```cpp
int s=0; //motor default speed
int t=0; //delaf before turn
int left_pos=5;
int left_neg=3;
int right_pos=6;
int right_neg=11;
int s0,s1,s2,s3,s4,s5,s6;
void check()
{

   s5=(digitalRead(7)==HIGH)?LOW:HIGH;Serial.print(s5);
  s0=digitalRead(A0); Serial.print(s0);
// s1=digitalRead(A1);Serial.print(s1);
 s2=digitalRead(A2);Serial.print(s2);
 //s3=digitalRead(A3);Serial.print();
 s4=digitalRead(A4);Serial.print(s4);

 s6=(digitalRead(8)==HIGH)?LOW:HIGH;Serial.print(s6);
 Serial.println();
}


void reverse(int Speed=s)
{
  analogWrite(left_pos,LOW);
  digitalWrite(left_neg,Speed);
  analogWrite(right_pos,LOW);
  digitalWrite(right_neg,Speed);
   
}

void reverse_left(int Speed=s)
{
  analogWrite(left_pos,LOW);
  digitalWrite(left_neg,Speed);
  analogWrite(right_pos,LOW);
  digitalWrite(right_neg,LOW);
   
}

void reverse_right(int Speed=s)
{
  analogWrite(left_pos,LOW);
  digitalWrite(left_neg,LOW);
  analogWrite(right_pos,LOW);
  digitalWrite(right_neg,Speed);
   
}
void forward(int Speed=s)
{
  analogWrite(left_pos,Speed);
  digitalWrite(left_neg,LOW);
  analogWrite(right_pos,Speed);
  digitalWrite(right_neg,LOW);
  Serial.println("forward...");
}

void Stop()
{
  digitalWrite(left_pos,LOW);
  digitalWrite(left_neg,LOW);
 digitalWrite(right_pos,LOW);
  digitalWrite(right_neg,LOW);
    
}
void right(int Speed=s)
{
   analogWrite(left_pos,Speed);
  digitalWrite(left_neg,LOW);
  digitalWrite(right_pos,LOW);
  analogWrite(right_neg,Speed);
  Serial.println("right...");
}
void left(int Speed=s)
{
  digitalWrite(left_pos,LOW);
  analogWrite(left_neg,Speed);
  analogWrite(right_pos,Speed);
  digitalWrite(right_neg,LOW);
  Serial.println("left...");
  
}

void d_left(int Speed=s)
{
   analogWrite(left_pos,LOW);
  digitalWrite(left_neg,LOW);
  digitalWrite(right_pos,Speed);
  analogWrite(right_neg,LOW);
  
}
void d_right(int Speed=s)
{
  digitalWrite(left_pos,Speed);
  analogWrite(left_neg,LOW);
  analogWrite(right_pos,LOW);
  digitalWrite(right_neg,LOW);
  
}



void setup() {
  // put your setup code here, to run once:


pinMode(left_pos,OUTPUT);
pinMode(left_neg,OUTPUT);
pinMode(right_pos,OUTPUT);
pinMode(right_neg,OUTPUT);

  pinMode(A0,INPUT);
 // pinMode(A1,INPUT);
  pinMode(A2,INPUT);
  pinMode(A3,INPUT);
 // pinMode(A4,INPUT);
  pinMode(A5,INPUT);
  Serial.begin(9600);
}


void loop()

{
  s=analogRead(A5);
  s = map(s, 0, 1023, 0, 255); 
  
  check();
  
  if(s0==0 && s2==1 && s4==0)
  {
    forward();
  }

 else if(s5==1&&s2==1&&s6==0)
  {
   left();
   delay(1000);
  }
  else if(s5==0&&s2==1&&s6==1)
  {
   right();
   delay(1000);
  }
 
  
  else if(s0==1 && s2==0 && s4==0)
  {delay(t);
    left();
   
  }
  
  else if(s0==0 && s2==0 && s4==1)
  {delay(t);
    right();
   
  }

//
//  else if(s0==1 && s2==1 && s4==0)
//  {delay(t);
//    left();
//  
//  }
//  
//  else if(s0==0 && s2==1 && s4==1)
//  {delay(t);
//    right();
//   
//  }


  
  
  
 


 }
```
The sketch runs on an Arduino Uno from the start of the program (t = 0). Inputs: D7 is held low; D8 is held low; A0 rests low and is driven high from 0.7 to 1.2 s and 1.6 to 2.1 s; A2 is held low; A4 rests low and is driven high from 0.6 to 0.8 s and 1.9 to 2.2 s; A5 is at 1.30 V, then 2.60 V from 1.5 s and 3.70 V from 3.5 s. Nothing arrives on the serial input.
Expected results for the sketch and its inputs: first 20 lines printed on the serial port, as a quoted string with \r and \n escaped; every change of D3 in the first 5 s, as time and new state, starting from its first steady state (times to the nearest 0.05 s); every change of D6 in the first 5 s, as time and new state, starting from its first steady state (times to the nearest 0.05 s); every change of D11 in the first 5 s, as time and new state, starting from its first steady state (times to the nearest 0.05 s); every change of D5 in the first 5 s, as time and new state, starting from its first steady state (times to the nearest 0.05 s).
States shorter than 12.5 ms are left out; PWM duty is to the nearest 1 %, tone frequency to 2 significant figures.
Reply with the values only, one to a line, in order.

"10001\r\n10001\r\n10001\r\n10001\r\n10001\r\n10001\r\n10001\r\n10001\r\n10001\r\n10001\r\n10001\r\n10001\r\n10001\r\n10001\r\n10001\r\n10001\r\n10001\r\n10001\r\n10001\r\n10001\r\n"
0 s low; 0.8 s PWM 26 %; 1.6 s PWM 52 %; 2.1 s low
0 s low; 0.8 s PWM 26 %; 1.6 s PWM 52 %; 2.1 s low
0 s low; 0.6 s PWM 26 %; 0.8 s low; 2.1 s PWM 52 %
0 s low; 0.6 s PWM 26 %; 0.8 s low; 2.1 s PWM 52 %
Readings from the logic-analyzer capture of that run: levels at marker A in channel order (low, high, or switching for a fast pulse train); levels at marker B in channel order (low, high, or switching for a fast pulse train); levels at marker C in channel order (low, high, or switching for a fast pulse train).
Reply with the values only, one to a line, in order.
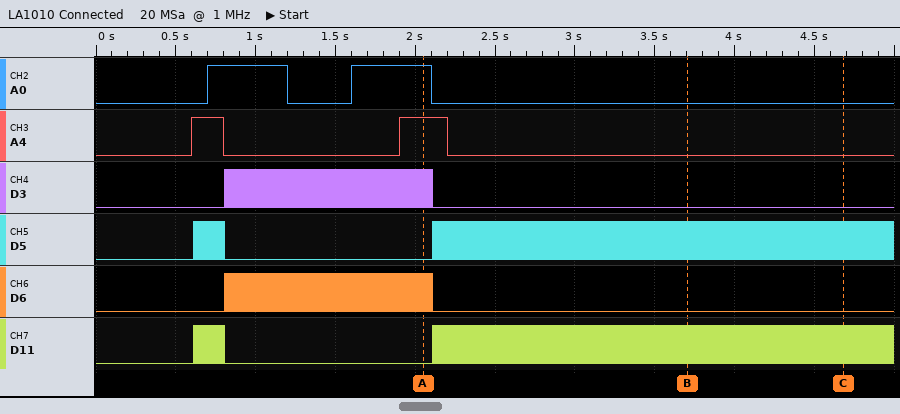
A0 high, A4 high, D3 switching, D5 low, D6 switching, D11 low
A0 low, A4 low, D3 low, D5 switching, D6 low, D11 switching
A0 low, A4 low, D3 low, D5 switching, D6 low, D11 switching
